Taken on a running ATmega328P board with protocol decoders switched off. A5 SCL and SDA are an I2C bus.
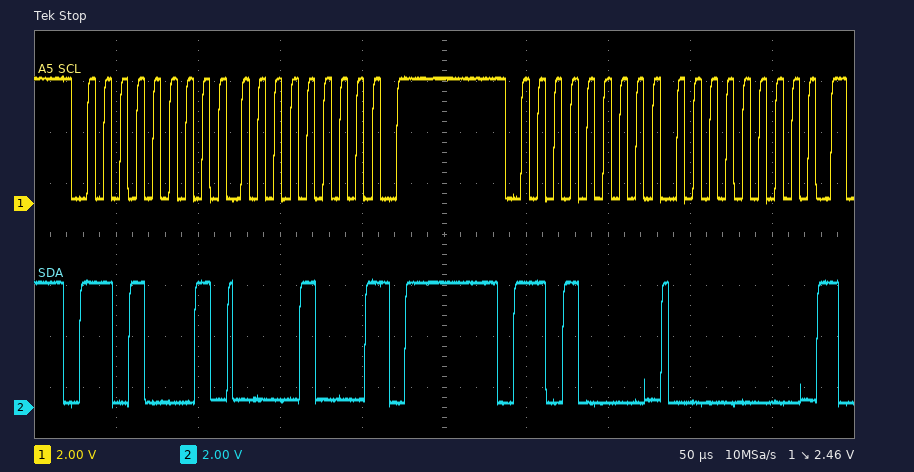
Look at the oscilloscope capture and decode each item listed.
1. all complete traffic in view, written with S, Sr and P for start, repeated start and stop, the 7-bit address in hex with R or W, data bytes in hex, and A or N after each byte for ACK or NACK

S 68R A 08 N P S 68W A 00 A
